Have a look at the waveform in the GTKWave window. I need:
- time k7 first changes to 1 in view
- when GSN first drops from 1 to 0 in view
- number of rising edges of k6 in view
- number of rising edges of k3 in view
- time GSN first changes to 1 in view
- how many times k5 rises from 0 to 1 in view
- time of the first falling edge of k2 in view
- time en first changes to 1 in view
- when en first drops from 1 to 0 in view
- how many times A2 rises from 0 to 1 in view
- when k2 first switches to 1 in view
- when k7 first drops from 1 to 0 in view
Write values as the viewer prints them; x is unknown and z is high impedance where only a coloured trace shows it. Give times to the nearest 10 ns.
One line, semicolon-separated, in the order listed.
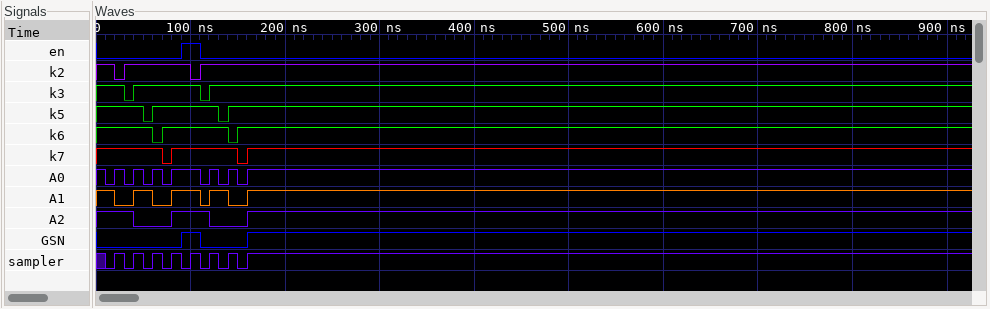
80 ns; 110 ns; 2; 2; 90 ns; 2; 20 ns; 90 ns; 110 ns; 2; 30 ns; 70 ns
